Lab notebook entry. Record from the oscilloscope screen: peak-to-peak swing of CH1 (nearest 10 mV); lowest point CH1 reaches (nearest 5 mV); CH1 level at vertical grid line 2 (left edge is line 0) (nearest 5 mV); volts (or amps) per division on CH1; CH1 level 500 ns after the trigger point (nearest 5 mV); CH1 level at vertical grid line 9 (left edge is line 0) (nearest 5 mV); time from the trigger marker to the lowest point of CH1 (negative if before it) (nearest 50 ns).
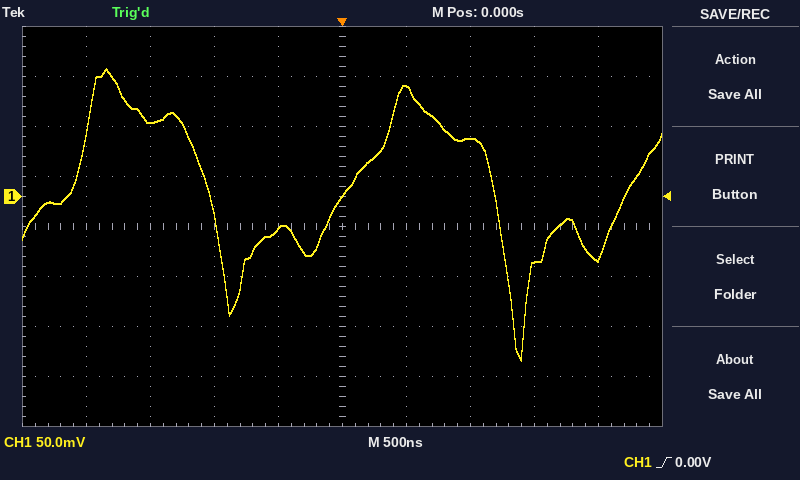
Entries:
290 mV
-165 mV
75 mV
50 mV
110 mV
-60 mV
+1.40 µs
